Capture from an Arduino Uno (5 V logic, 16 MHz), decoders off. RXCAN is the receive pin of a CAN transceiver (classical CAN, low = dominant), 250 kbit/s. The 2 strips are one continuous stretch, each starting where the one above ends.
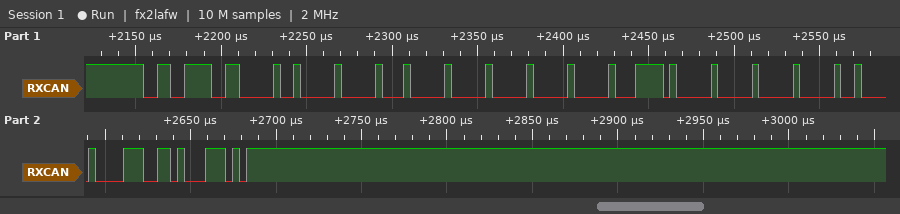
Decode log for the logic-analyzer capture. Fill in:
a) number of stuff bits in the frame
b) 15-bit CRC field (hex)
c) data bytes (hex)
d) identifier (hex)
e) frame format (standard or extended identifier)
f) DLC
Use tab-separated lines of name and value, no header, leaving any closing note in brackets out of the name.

number of stuff bits in the frame	12
15-bit CRC field	0x668E
data bytes	00 00 00 7A 00 00 04 21
identifier	0x0CF00400
frame format	extended
DLC	8
